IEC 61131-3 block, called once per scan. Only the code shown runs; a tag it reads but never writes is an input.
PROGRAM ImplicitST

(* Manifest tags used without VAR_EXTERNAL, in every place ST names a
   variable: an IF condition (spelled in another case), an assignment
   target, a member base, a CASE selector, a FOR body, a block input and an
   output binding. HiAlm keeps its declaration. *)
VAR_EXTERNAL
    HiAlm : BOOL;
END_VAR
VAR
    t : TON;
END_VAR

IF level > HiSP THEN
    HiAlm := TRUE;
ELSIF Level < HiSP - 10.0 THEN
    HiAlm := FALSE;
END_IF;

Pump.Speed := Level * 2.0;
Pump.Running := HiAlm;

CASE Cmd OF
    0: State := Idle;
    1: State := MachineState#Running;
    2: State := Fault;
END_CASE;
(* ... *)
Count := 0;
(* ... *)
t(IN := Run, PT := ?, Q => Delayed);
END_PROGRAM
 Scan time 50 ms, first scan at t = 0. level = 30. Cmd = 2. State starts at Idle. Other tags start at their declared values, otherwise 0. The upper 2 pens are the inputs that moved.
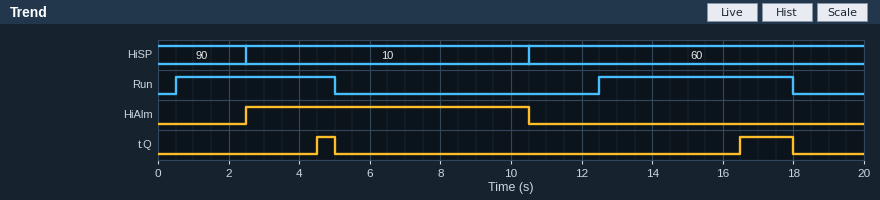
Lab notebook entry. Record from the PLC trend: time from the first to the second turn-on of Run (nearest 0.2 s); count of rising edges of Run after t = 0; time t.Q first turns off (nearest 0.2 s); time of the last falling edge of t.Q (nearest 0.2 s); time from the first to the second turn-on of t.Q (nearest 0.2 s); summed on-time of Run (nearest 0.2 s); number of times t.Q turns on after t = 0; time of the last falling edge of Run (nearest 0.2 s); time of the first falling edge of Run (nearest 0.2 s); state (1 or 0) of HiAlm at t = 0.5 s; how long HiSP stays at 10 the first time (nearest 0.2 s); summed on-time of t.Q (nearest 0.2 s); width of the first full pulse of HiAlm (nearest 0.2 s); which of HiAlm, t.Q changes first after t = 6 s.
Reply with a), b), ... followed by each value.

a) 12.0 s
b) 2
c) 5.0 s
d) 18.0 s
e) 12.0 s
f) 10.0 s
g) 2
h) 18.0 s
i) 5.0 s
j) 0
k) 8.0 s
l) 2.0 s
m) 8.0 s
n) HiAlm
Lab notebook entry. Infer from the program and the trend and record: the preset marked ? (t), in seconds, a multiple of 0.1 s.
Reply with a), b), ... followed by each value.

a) 4.0 s
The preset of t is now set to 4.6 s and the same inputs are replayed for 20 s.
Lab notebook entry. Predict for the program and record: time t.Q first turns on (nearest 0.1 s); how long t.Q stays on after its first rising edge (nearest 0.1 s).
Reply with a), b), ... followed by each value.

a) 17.1 s
b) 0.9 s
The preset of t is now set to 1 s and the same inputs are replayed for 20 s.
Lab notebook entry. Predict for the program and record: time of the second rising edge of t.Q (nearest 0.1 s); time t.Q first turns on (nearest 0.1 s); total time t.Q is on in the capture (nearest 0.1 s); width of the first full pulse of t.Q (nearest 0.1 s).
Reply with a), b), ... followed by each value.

a) 13.5 s
b) 1.5 s
c) 8.0 s
d) 3.5 s
